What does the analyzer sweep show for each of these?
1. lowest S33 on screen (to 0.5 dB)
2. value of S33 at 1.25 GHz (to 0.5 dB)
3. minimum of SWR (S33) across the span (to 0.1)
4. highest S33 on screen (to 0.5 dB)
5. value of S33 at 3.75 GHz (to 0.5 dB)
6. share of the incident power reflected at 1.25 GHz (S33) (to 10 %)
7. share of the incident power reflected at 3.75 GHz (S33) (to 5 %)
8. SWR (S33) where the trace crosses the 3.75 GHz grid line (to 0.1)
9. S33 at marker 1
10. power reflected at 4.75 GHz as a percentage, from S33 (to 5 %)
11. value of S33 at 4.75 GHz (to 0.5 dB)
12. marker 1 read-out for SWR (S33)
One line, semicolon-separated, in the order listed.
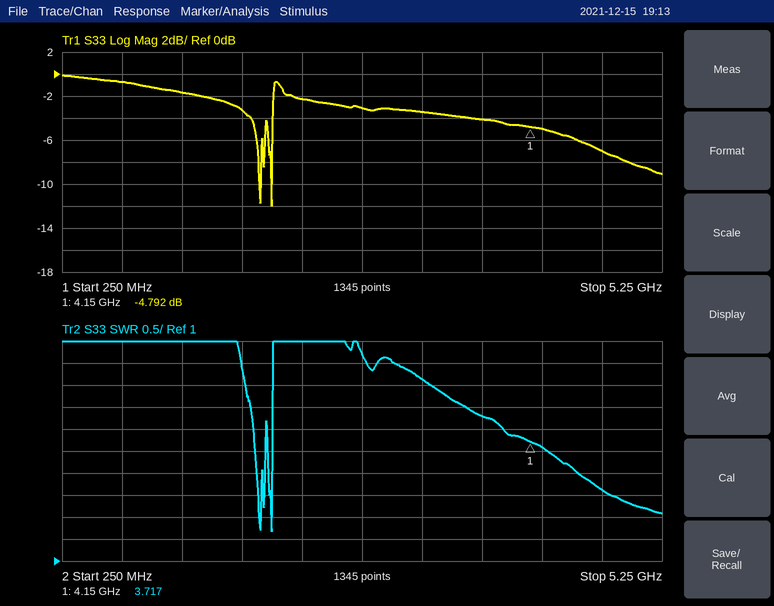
-12.0 dB; -1.5 dB; 1.7; 0.0 dB; -4.0 dB; 70 %; 40 %; 4.3; -4.792 dB; 20 %; -7.0 dB; 3.717
